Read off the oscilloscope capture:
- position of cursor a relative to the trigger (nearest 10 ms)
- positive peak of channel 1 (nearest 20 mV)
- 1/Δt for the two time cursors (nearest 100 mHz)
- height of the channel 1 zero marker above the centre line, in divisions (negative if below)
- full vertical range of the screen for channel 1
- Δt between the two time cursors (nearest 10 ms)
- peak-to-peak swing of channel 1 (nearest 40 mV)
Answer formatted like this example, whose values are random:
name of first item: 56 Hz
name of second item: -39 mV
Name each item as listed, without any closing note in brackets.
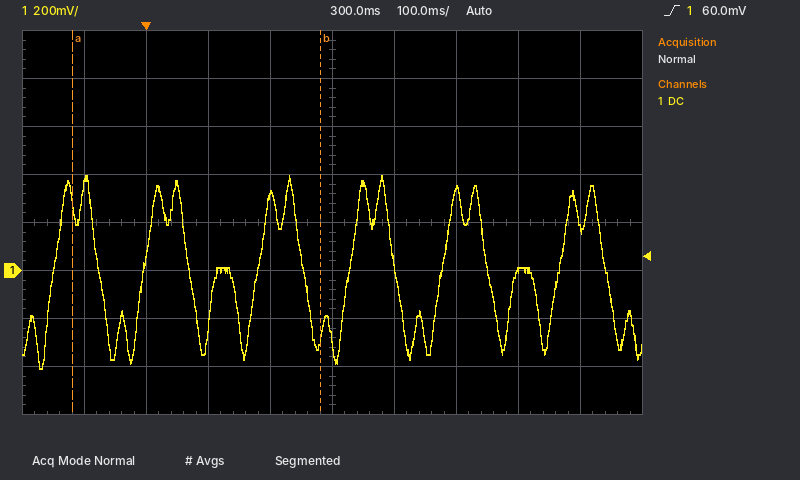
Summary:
position of cursor a relative to the trigger: -120 ms
positive peak of channel 1: 400 mV
1/Δt for the two time cursors: 2.5 Hz
height of the channel 1 zero marker above the centre line, in divisions: -1.0 div
full vertical range of the screen for channel 1: 1.6 V
Δt between the two time cursors: 400 ms
peak-to-peak swing of channel 1: 800 mV
